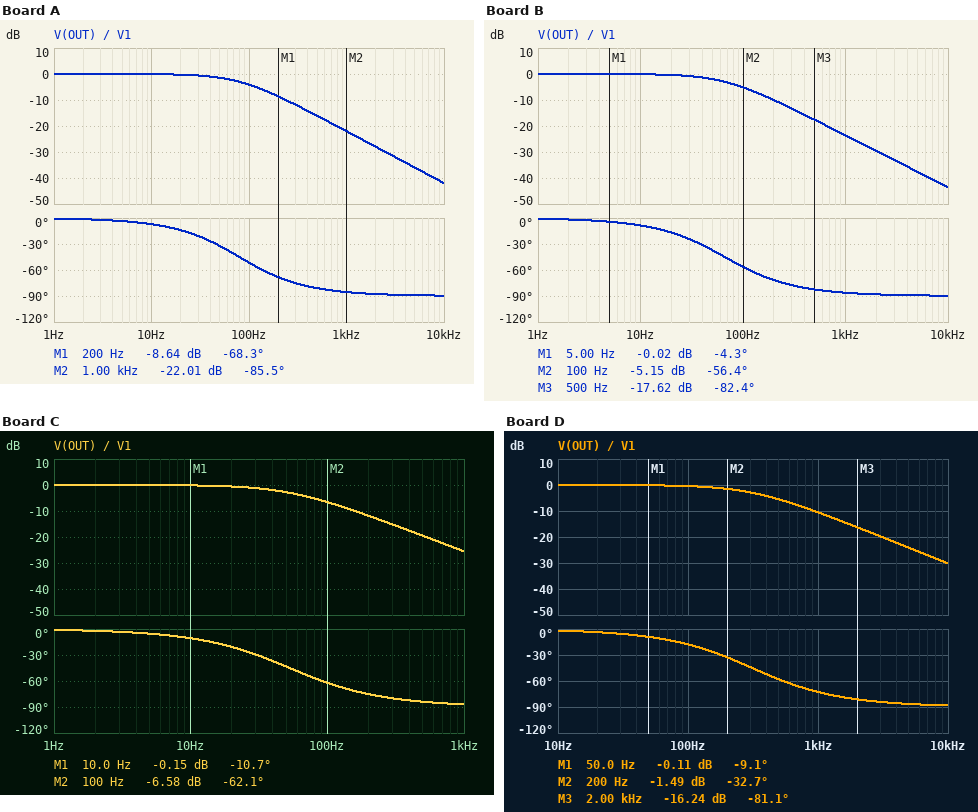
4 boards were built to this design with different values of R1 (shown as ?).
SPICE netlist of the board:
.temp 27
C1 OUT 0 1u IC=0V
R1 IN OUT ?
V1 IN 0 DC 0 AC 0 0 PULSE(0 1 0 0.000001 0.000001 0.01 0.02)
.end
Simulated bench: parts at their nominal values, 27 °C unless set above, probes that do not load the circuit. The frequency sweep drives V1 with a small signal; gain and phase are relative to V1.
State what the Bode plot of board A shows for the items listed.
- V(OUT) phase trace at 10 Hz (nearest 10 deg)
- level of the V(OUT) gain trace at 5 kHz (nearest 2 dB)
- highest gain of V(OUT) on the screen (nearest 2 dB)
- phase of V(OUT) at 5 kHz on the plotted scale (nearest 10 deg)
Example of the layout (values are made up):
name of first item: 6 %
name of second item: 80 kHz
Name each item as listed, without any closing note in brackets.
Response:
V(OUT) phase trace at 10 Hz: -10 deg
level of the V(OUT) gain trace at 5 kHz: -36 dB
highest gain of V(OUT) on the screen: 0 dB
phase of V(OUT) at 5 kHz on the plotted scale: -90 deg
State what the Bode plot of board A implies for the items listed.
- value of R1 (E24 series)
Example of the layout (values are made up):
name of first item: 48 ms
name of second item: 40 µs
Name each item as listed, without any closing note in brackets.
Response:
value of R1: 2 kΩ
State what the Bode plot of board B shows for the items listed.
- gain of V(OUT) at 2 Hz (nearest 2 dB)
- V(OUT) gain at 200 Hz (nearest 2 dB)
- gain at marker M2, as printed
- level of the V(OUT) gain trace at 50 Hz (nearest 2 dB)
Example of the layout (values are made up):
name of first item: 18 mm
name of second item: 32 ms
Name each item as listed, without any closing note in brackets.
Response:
gain of V(OUT) at 2 Hz: 0 dB
V(OUT) gain at 200 Hz: -10 dB
gain at marker M2, as printed: -5.15 dB
level of the V(OUT) gain trace at 50 Hz: -2 dB
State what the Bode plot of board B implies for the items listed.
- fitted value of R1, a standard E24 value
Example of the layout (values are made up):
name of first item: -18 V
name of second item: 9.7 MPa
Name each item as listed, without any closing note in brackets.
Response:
fitted value of R1, a standard E24 value: 2.4 kΩ
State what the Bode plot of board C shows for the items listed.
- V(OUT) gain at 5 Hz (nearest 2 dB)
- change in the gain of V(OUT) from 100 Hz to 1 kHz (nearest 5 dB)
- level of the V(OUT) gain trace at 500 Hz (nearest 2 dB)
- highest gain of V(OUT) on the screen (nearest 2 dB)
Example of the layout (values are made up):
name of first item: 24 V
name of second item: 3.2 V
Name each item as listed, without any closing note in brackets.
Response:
V(OUT) gain at 5 Hz: 0 dB
change in the gain of V(OUT) from 100 Hz to 1 kHz: -20 dB
level of the V(OUT) gain trace at 500 Hz: -20 dB
highest gain of V(OUT) on the screen: 0 dB
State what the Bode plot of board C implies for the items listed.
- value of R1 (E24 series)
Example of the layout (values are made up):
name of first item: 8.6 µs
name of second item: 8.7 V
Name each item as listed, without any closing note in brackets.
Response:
value of R1: 3 kΩ
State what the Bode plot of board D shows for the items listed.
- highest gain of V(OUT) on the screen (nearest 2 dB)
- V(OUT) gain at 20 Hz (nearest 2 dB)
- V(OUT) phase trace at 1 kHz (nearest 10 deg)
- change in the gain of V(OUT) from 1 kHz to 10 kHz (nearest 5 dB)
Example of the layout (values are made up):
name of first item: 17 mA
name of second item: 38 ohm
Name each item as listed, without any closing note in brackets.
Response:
highest gain of V(OUT) on the screen: 0 dB
V(OUT) gain at 20 Hz: 0 dB
V(OUT) phase trace at 1 kHz: -70 deg
change in the gain of V(OUT) from 1 kHz to 10 kHz: -20 dB
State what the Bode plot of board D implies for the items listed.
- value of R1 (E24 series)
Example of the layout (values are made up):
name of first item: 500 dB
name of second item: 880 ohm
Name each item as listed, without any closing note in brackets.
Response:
value of R1: 510 Ω
